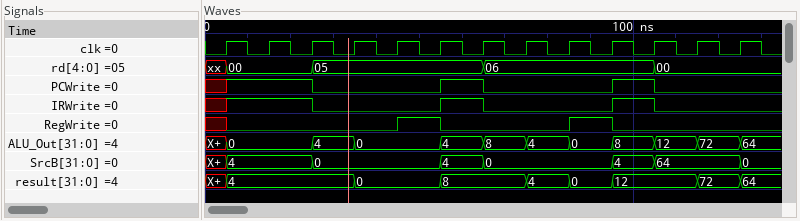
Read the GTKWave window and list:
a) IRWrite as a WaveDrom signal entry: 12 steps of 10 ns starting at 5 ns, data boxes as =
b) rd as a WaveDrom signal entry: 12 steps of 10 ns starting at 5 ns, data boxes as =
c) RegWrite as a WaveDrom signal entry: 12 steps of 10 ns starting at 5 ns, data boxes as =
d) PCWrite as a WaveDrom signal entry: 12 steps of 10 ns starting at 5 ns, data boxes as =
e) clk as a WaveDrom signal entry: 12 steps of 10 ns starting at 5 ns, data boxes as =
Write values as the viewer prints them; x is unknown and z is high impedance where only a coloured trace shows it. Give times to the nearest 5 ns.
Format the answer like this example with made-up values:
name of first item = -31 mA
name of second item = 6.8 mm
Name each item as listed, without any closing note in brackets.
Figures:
IRWrite as a WaveDrom signal entry: 12 steps of 10 ns starting at 5 ns, data boxes as = = {name: 'IRWrite', wave: '1.0..10..10.'}
rd as a WaveDrom signal entry: 12 steps of 10 ns starting at 5 ns, data boxes as = = {name: 'rd', wave: '=.=...=...=.', data: '00 05 06 00'}
RegWrite as a WaveDrom signal entry: 12 steps of 10 ns starting at 5 ns, data boxes as = = {name: 'RegWrite', wave: '0...10..10..'}
PCWrite as a WaveDrom signal entry: 12 steps of 10 ns starting at 5 ns, data boxes as = = {name: 'PCWrite', wave: '1.0..10..10.'}
clk as a WaveDrom signal entry: 12 steps of 10 ns starting at 5 ns, data boxes as = = {name: 'clk', wave: 'p...........'}
